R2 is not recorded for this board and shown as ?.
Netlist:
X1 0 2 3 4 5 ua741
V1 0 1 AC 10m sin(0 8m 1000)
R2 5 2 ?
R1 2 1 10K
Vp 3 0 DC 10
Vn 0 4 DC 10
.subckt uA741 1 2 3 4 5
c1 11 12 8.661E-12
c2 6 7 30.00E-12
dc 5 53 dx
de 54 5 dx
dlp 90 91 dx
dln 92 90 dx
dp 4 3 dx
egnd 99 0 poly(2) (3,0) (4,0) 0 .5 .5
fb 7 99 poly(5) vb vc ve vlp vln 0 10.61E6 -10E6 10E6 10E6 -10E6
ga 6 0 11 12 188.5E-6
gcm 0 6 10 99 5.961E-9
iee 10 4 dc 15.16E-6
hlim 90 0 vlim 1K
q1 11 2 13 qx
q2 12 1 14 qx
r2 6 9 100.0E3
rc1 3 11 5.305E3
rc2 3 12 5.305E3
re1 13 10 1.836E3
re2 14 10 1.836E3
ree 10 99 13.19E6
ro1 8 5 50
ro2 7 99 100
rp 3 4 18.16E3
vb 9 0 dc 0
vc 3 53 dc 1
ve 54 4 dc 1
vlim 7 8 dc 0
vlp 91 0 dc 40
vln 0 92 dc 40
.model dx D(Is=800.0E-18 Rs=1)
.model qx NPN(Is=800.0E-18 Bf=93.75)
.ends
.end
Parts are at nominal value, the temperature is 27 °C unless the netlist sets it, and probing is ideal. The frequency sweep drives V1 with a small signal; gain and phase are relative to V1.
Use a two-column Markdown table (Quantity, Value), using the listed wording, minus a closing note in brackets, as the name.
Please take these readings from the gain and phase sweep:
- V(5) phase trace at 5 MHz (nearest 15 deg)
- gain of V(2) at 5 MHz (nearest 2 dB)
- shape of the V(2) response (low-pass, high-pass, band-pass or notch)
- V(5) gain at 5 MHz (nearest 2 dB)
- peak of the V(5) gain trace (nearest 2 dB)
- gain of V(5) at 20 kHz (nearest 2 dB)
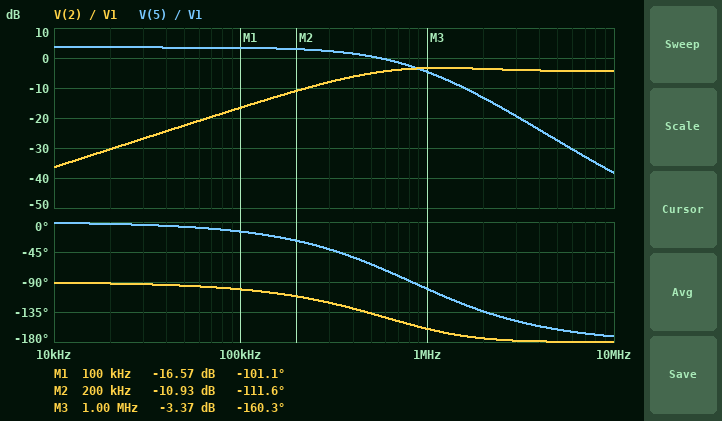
| Quantity | Value |
|---|---|
| V(5) phase trace at 5 MHz | -165 deg |
| gain of V(2) at 5 MHz | -4 dB |
| shape of the V(2) response | high-pass |
| V(5) gain at 5 MHz | -28 dB |
| peak of the V(5) gain trace | 4 dB |
| gain of V(5) at 20 kHz | 4 dB |
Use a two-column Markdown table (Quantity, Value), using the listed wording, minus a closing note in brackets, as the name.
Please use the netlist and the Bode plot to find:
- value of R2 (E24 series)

| Quantity | Value |
|---|---|
| value of R2 | 15 kΩ |
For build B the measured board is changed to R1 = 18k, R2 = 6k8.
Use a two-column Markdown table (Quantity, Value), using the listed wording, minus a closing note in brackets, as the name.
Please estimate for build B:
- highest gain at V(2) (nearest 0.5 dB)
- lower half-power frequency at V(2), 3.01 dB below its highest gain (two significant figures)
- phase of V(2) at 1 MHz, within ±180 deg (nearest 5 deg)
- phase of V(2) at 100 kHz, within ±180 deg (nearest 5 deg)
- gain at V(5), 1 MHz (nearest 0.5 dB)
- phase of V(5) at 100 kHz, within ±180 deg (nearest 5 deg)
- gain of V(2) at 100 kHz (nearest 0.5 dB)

| Quantity | Value |
|---|---|
| highest gain at V(2) | -9.5 dB |
| lower half-power frequency at V(2), 3.01 dB below its highest gain | 660 kHz |
| phase of V(2) at 1 MHz, within ±180 deg | -140 deg |
| phase of V(2) at 100 kHz, within ±180 deg | -95 deg |
| gain at V(5), 1 MHz | -11.5 dB |
| phase of V(5) at 100 kHz, within ±180 deg | -10 deg |
| gain of V(2) at 100 kHz | -28.5 dB |
